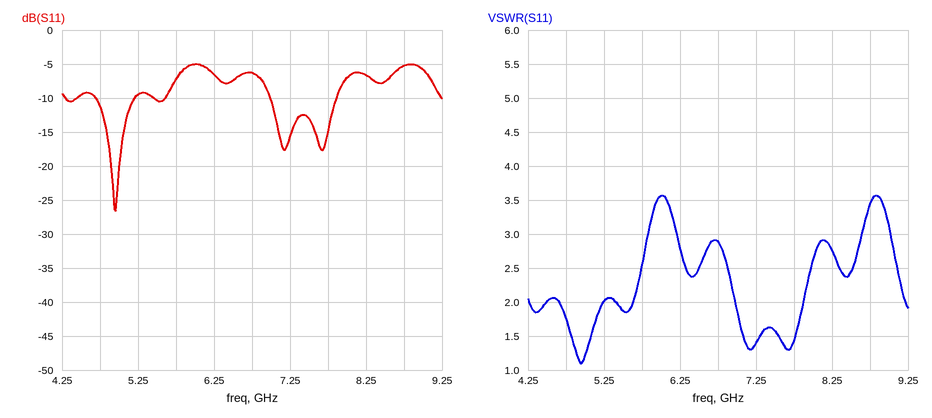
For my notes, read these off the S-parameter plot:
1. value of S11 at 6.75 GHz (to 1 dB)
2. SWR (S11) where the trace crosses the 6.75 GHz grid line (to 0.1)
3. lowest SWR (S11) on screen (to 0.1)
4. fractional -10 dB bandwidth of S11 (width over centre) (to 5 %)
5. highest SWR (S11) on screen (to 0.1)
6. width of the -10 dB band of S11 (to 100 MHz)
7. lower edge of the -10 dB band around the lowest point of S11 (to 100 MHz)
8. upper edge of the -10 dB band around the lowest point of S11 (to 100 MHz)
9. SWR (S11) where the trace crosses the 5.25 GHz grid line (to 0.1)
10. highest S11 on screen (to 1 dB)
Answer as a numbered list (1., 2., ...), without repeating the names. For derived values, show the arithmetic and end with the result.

1. -6 dB
2. 2.9
3. 1.1
4. 500 MHz / 4.95 GHz ≈ 10 %
5. 3.6
6. 5.2 GHz − 4.7 GHz = 500 MHz
7. 4.7 GHz
8. 5.2 GHz
9. 2.0
10. -5 dB
